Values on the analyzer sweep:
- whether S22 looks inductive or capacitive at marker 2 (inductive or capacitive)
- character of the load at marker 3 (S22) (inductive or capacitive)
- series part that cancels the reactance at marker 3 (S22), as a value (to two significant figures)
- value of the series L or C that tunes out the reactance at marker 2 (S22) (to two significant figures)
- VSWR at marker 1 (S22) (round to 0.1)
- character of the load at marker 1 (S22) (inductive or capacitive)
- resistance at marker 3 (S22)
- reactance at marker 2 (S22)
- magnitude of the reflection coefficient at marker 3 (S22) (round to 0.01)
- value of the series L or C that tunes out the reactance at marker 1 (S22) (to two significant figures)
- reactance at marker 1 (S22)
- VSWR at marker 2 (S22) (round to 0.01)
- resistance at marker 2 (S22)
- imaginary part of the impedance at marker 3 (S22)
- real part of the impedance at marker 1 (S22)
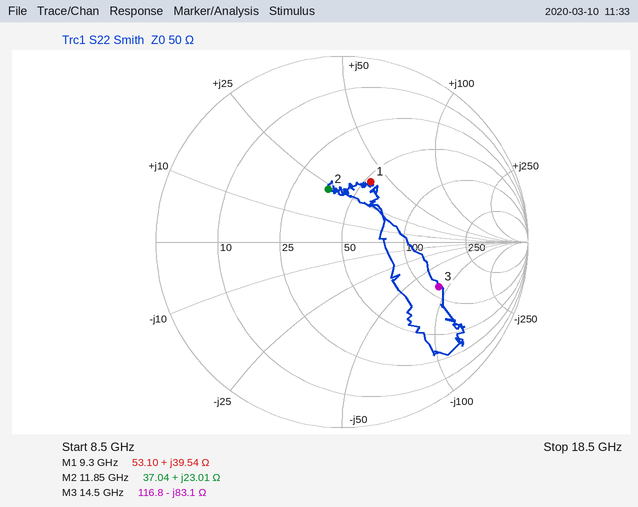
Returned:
inductive
capacitive
910 pH
580 fF
2.1
inductive
116.8 Ω
+23.01 Ω
0.57
430 fF
+39.54 Ω
1.83
37.04 Ω
-83.1 Ω
53.10 Ω
